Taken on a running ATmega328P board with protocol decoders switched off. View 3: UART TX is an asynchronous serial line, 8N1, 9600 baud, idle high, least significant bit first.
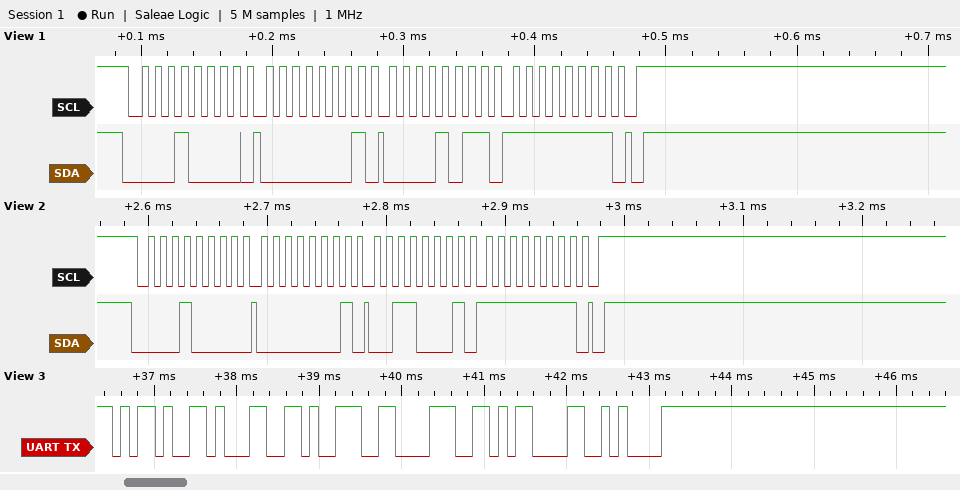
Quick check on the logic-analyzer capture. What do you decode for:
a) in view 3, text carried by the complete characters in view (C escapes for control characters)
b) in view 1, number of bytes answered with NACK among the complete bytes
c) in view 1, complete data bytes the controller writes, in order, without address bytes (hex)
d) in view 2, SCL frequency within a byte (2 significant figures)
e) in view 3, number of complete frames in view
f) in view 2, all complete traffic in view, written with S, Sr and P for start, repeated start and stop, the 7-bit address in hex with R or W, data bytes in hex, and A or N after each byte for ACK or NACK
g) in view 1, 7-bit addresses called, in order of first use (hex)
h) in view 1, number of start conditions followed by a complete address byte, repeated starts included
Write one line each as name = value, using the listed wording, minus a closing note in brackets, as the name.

in view 3, text carried by the complete characters in view = "-198\r\n"
in view 1, number of bytes answered with NACK among the complete bytes = 0
in view 1, complete data bytes the controller writes, in order, without address bytes = 01 0B FF
in view 2, SCL frequency within a byte = 100 kHz
in view 3, number of complete frames in view = 6
in view 2, all complete traffic in view, written with S, Sr and P for start, repeated start and stop, the 7-bit address in hex with R or W, data bytes in hex, and A or N after each byte for ACK or NACK = S 08W A 01 A 31 A FF A P
in view 1, 7-bit addresses called, in order of first use = 0x08
in view 1, number of start conditions followed by a complete address byte, repeated starts included = 1
